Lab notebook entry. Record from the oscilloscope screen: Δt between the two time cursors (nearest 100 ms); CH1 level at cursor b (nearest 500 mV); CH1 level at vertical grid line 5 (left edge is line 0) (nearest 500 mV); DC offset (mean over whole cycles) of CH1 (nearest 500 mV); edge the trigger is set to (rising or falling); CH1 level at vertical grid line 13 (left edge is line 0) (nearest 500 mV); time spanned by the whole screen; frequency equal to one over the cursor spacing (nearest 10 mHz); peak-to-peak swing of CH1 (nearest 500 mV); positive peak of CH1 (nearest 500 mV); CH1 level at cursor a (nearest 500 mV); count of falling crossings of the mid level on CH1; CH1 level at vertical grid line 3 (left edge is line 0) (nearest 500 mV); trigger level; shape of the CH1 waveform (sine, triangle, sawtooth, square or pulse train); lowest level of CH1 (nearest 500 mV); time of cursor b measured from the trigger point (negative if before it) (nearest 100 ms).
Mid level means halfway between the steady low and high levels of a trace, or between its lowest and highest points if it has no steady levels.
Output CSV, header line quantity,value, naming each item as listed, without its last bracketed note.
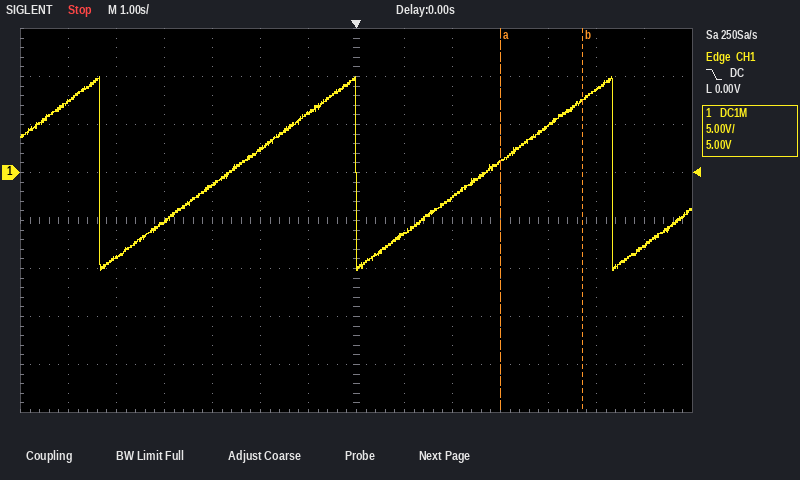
quantity,value
Δt between the two time cursors,1.7 s
CH1 level at cursor b,7.5 V
CH1 level at vertical grid line 5 (left edge is line 0),2.5 V
DC offset (mean over whole cycles) of CH1,0.0 V
edge the trigger is set to,falling
CH1 level at vertical grid line 13 (left edge is line 0),-7.5 V
time spanned by the whole screen,14 s
frequency equal to one over the cursor spacing,590 mHz
peak-to-peak swing of CH1,20.0 V
positive peak of CH1,10.0 V
CH1 level at cursor a,1.0 V
count of falling crossings of the mid level on CH1,3
CH1 level at vertical grid line 3 (left edge is line 0),-5.0 V
trigger level,0.00 V
shape of the CH1 waveform,sawtooth
lowest level of CH1,-10.0 V
time of cursor b measured from the trigger point (negative if before it),+4.7 s
